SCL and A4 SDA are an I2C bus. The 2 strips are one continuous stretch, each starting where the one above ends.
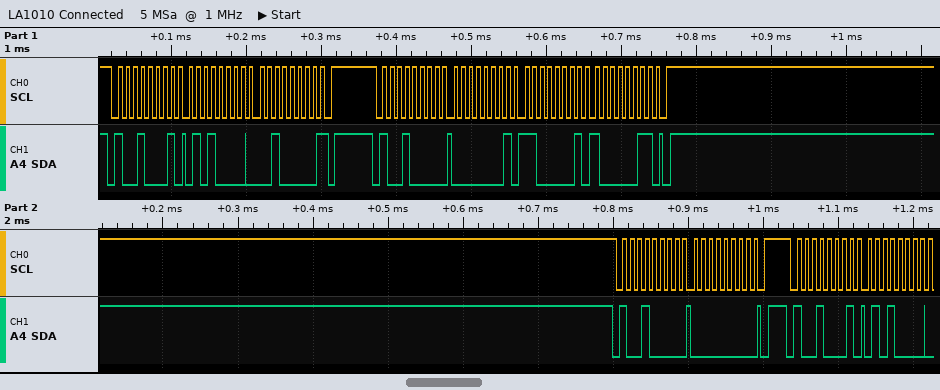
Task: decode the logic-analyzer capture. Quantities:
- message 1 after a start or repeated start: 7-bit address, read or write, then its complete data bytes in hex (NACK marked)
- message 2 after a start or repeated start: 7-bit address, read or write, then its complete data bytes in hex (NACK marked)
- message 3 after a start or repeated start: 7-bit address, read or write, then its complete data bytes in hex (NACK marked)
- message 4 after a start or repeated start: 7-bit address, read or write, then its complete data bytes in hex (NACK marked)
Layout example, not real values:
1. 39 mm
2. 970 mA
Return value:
1. 0x48 read: 50 20 NACK
2. 0x48 write: 01 C1 83
3. 0x48 write: 00
4. 0x48 read: 50
